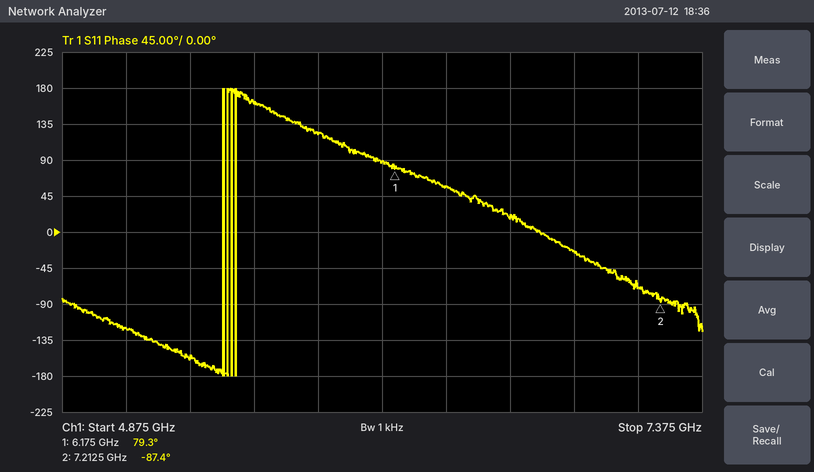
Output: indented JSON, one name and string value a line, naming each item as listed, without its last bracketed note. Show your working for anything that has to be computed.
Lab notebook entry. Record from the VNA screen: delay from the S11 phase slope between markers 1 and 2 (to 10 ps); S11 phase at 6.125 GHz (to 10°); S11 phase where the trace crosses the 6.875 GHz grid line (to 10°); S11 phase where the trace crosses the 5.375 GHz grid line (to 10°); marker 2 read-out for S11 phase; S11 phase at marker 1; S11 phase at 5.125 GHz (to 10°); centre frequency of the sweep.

{
  "delay from the S11 phase slope between markers 1 and 2": "−(-87.4° − (79.3°))/(360° × 1.0375 GHz) ≈ 446 ps, so 450 ps to the nearest 10 ps",
  "S11 phase at 6.125 GHz": "90°",
  "S11 phase where the trace crosses the 6.875 GHz grid line": "-20°",
  "S11 phase where the trace crosses the 5.375 GHz grid line": "-160°",
  "marker 2 read-out for S11 phase": "-87.4°",
  "S11 phase at marker 1": "79.3°",
  "S11 phase at 5.125 GHz": "-120°",
  "centre frequency of the sweep": "6.125 GHz"
}
